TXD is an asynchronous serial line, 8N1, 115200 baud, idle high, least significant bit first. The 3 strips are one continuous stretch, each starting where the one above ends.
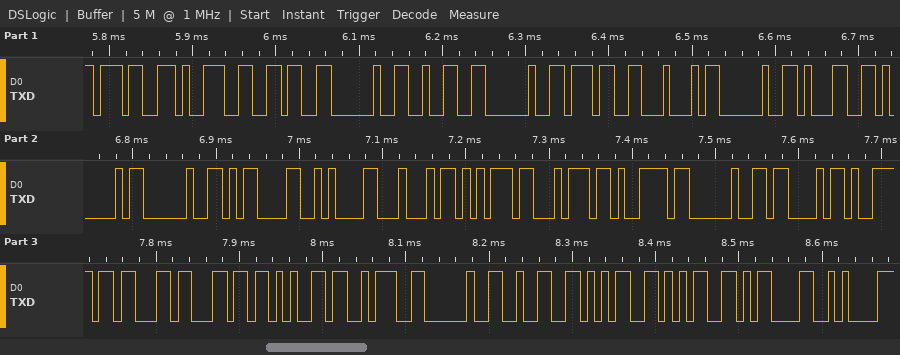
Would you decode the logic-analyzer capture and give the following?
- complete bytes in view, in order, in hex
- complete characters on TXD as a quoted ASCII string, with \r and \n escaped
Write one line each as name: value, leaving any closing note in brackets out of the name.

complete bytes in view, in order, in hex: 0x37 0x39 0x36 0x20 0x32 0x20 0x37 0x44 0x20 0x31 0x41 0x20 0x0D 0x0A 0x44 0x75 0x74 0x79 0x20 0x43 0x79 0x63 0x6C 0x65 0x3A 0x20 0x32 0x35 0x35 0x0D 0x0A
complete characters on TXD as a quoted ASCII string, with \r and \n escaped: "796 2 7D 1A \r\nDuty Cycle: 255\r\n"
